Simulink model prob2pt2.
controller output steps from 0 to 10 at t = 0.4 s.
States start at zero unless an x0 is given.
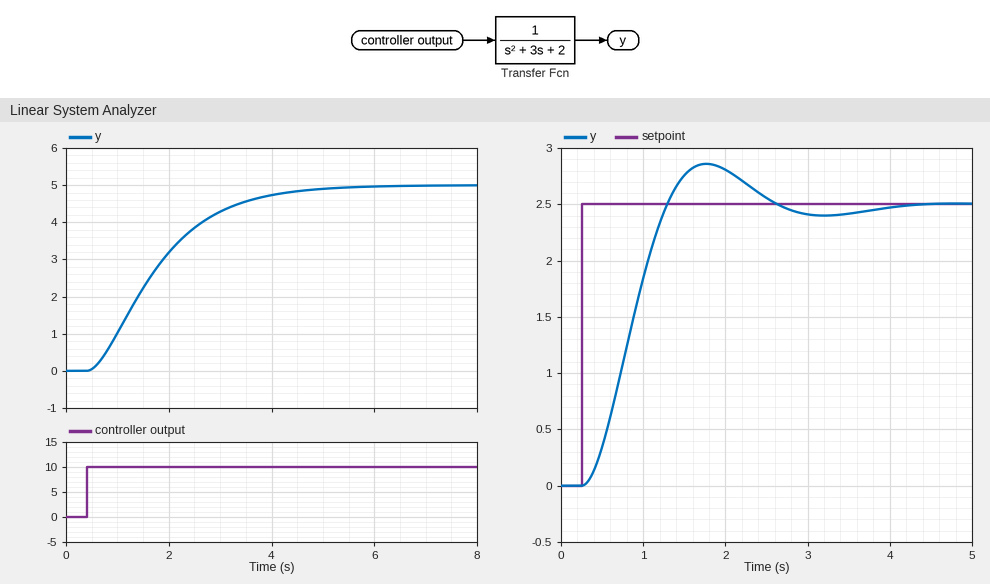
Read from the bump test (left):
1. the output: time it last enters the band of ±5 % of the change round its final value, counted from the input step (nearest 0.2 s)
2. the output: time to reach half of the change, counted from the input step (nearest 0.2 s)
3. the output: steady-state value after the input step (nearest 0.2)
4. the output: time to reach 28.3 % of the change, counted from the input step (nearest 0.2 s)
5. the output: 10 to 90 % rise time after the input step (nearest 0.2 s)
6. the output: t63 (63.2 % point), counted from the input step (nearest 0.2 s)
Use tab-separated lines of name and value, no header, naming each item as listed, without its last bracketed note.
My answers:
the output: time it last enters the band of ±5 % of the change round its final value, counted from the input step	3.6 s
the output: time to reach half of the change, counted from the input step	1.2 s
the output: steady-state value after the input step	5.0
the output: time to reach 28.3 % of the change, counted from the input step	0.8 s
the output: 10 to 90 % rise time after the input step	2.6 s
the output: t63 (63.2 % point), counted from the input step	1.6 s
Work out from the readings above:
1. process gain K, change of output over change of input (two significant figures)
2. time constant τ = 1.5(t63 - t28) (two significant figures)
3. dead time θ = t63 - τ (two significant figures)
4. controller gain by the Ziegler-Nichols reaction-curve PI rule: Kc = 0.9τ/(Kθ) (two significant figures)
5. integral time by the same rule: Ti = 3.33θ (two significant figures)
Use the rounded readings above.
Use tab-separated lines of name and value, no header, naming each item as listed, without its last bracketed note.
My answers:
process gain K, change of output over change of input	0.50
time constant τ = 1.5(t63 - t28)	1.2 s
dead time θ = t63 - τ	0.40 s
controller gain by the Ziegler-Nichols reaction-curve PI rule: Kc = 0.9τ/(Kθ)	5.4
integral time by the same rule: Ti = 3.33θ	1.3 s
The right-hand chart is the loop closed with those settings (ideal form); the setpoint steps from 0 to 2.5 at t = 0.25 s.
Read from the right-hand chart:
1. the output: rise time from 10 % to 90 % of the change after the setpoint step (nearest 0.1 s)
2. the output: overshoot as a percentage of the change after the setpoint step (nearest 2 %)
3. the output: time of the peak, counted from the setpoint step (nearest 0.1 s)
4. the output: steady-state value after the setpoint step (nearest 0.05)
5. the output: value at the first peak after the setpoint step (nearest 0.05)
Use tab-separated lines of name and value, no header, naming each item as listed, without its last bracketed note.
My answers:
the output: rise time from 10 % to 90 % of the change after the setpoint step	0.7 s
the output: overshoot as a percentage of the change after the setpoint step	14 %
the output: time of the peak, counted from the setpoint step	1.5 s
the output: steady-state value after the setpoint step	2.50
the output: value at the first peak after the setpoint step	2.85
